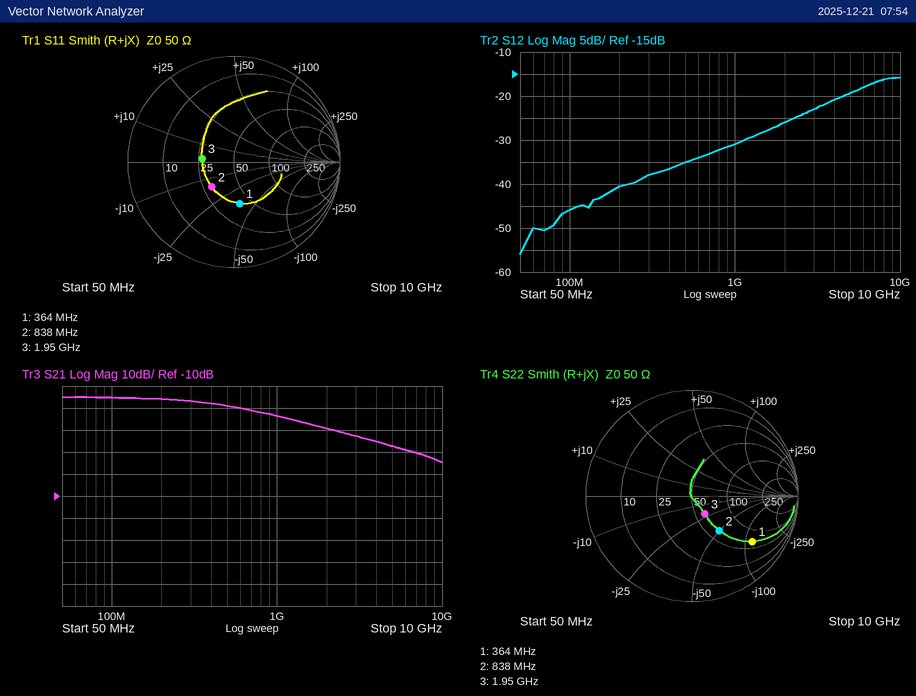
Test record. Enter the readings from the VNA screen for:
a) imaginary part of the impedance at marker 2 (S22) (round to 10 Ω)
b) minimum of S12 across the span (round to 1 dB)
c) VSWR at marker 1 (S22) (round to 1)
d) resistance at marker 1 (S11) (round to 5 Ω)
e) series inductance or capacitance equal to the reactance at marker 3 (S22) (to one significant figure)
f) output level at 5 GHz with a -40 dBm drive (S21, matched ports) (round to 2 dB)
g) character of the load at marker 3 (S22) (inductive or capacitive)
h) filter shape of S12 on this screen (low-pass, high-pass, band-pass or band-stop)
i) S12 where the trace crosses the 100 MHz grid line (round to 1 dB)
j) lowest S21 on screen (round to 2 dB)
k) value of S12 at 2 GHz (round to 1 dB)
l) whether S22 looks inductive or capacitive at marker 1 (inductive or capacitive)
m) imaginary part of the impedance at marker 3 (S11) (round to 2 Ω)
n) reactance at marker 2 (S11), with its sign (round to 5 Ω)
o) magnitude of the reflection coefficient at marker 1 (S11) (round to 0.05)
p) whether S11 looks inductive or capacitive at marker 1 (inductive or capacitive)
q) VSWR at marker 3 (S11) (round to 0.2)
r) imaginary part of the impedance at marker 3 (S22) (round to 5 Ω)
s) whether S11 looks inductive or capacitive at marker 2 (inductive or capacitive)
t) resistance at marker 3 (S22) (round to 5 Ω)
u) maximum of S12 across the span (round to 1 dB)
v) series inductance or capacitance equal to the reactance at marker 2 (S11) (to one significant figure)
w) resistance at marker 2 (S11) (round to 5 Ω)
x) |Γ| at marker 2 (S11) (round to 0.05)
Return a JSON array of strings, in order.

["-50 Ω", "-56 dB", "6", "40 Ω", "4 pF", "-28 dBm", "capacitive", "high-pass", "-46 dB", "6 dB", "-26 dB", "capacitive", "+2 Ω", "-15 Ω", "0.40", "capacitive", "1.8", "-20 Ω", "capacitive", "60 Ω", "-16 dB", "10 pF", "30 Ω", "0.30"]
